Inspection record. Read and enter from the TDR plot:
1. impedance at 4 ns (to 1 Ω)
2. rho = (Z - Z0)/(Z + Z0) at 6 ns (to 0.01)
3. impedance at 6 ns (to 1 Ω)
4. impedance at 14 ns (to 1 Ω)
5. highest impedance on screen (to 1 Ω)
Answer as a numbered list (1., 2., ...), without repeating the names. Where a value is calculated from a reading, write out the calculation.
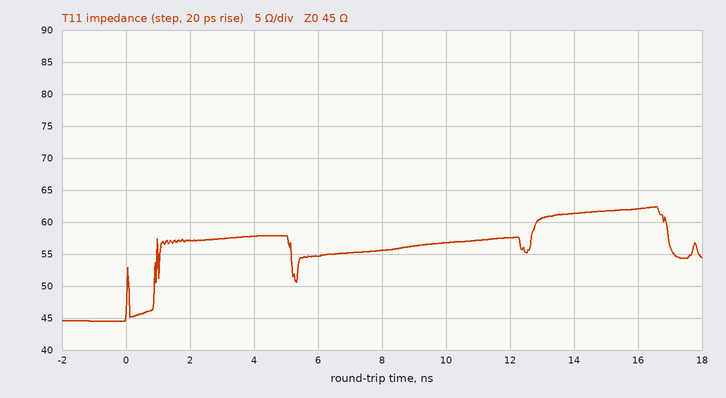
1. 58 Ω
2. (55 − 45)/(55 + 45) ≈ +0.10
3. 55 Ω
4. 61 Ω
5. 62 Ω
